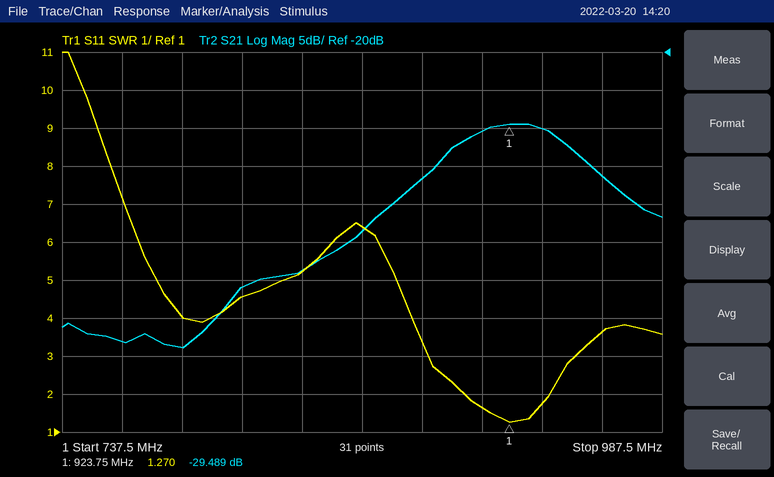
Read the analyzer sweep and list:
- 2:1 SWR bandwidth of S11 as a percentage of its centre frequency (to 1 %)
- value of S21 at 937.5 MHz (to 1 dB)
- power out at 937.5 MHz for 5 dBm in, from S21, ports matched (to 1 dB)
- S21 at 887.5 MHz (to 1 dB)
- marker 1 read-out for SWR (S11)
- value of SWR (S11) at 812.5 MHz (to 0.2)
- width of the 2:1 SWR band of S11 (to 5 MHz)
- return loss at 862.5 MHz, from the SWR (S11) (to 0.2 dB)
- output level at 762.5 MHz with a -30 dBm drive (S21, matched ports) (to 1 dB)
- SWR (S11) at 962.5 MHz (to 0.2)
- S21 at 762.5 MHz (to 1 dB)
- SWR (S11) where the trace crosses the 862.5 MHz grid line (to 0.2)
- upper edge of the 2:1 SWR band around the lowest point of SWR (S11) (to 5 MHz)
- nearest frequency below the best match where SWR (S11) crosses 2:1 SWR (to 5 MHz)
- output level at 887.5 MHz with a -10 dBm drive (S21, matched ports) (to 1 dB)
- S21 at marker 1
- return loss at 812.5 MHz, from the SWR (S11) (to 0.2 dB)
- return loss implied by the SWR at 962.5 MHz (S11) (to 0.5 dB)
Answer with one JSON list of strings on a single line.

["4 %", "-30 dB", "-25 dBm", "-37 dB", "1.270", "4.6", "35 MHz", "2.8 dB", "-88 dBm", "3.6", "-58 dB", "6.4", "940 MHz", "905 MHz", "-47 dBm", "-29.489 dB", "3.8 dB", "5.0 dB"]
